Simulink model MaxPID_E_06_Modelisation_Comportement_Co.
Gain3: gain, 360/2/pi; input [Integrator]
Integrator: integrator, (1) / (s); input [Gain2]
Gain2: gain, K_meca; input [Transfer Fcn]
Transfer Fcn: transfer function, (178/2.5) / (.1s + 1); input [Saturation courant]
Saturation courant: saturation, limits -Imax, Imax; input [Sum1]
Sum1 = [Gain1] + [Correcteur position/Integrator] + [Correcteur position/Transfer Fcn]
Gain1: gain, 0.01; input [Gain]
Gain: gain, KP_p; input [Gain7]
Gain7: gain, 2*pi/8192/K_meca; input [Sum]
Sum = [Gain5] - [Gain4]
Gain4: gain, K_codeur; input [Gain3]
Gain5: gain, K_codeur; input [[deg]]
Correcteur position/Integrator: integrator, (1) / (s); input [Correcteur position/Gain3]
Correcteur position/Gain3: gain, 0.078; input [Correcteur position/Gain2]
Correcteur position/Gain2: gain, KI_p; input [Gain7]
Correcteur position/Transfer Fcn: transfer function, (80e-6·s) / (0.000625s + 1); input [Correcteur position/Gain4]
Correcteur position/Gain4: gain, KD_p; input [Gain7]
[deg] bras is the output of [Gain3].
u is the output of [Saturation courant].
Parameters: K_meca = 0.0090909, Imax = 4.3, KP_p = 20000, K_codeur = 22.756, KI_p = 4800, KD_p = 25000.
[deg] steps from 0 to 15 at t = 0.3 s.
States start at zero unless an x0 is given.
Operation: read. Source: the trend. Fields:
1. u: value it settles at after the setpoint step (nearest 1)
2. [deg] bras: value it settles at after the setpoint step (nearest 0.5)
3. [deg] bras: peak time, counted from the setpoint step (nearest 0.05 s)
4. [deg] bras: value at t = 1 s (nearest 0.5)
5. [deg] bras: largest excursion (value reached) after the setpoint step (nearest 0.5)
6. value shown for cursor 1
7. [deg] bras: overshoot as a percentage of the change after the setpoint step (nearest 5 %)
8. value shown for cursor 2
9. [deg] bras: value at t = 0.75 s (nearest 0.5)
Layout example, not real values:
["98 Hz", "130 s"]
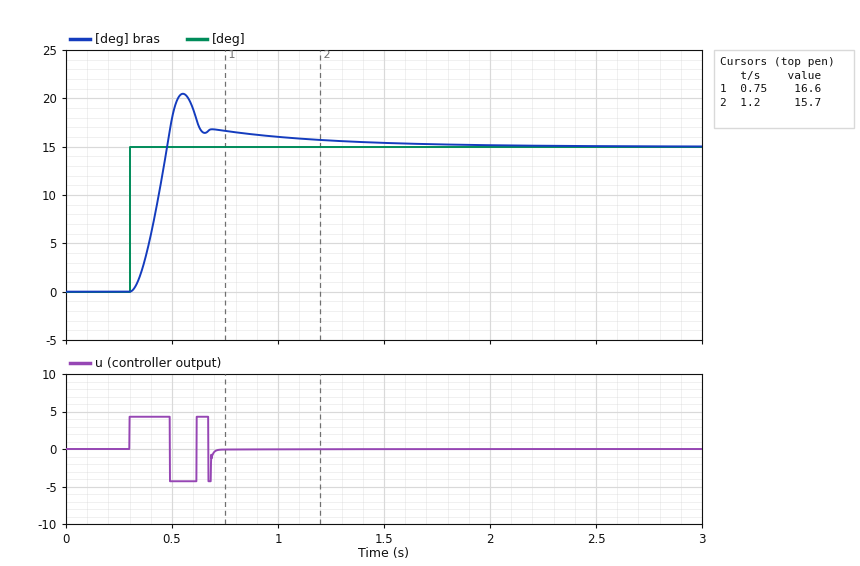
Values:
["0", "15.0", "0.25 s", "16.0", "20.5", "16.6", "35 %", "15.7", "16.5"]
